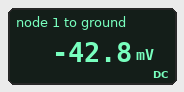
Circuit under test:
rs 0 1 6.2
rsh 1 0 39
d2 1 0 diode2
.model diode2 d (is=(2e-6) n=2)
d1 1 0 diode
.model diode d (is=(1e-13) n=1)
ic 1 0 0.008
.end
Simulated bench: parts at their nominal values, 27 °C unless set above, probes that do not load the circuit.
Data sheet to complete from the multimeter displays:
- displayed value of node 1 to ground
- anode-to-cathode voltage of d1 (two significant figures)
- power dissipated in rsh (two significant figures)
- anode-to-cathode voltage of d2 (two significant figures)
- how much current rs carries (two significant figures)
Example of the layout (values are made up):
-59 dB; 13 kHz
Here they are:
-42.8 mV; -43 mV; 47 µW; -43 mV; 6.9 mA
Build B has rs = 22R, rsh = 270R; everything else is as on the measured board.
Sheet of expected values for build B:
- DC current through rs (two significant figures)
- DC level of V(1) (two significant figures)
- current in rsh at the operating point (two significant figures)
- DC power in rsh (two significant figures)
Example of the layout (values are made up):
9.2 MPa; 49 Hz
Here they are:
7.4 mA; -160 mV; 600 µA; 98 µW
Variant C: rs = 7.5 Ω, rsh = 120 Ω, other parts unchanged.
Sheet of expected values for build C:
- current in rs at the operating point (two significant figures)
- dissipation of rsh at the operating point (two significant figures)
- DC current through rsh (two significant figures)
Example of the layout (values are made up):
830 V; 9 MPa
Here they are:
7.5 mA; 27 µW; 470 µA
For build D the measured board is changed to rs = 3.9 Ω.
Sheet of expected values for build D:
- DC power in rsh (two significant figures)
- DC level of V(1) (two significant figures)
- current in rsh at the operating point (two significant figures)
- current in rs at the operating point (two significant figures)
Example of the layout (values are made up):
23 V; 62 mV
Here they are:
21 µW; -28 mV; 730 µA; 7.3 mA
